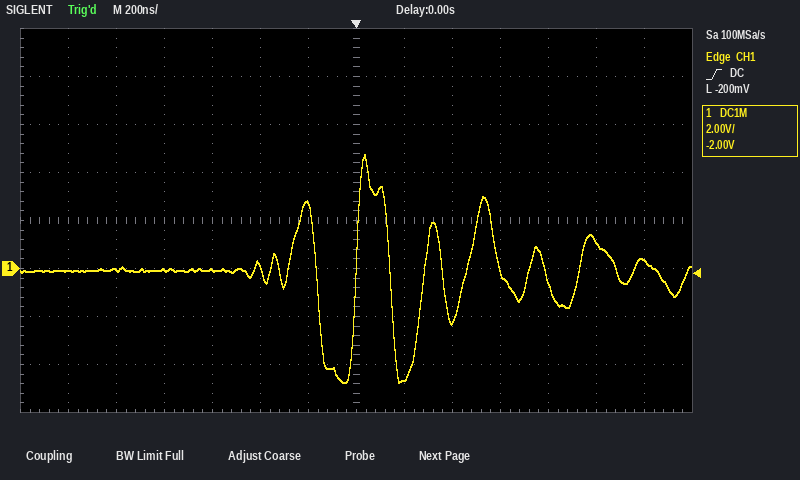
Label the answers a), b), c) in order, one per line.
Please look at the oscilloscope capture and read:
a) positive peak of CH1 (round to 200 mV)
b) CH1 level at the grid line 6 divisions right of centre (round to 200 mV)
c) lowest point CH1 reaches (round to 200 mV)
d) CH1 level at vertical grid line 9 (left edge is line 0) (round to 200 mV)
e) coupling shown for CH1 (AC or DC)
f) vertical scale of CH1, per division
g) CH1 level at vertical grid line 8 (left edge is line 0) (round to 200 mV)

a) 4.8 V
b) 400 mV
c) -4.8 V
d) -2.2 V
e) DC
f) 2 V
g) -4.6 V
